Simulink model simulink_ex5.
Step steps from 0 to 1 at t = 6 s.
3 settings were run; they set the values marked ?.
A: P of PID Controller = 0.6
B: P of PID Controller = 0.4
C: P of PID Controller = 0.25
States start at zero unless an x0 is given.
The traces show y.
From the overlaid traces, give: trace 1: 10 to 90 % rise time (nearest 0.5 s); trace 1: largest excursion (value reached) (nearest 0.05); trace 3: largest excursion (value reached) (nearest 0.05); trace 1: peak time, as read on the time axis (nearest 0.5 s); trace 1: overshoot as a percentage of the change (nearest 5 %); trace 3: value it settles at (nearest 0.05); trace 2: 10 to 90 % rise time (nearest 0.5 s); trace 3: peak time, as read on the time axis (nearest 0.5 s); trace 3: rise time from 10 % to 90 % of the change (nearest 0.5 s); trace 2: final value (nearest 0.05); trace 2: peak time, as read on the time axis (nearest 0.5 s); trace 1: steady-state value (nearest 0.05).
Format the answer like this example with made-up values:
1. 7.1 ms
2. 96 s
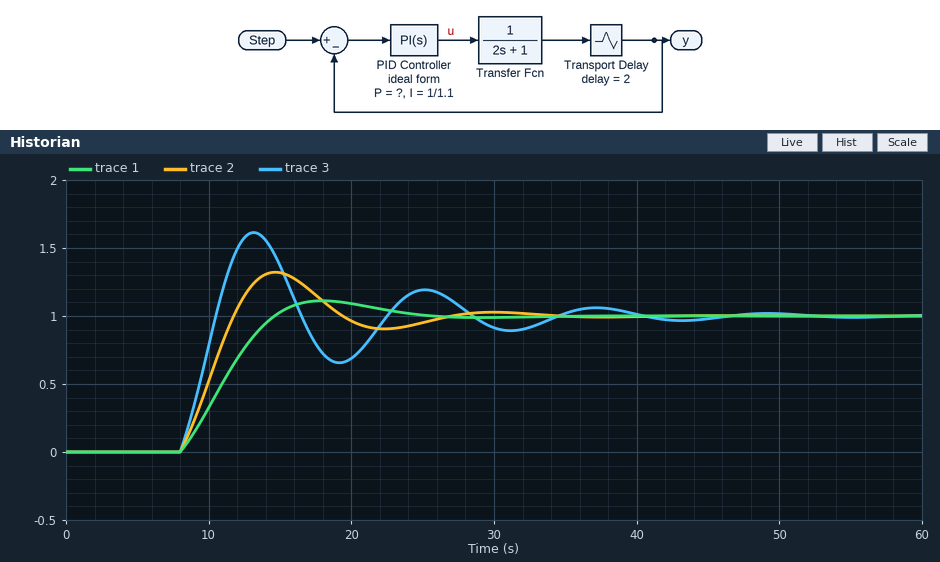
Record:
1. 5.0 s
2. 1.10
3. 1.60
4. 18.0 s
5. 10 %
6. 1.00
7. 3.0 s
8. 13.0 s
9. 2.0 s
10. 1.00
11. 14.5 s
12. 1.00
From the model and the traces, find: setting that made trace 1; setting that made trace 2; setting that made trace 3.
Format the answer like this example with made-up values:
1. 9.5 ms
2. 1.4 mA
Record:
1. C
2. B
3. A
